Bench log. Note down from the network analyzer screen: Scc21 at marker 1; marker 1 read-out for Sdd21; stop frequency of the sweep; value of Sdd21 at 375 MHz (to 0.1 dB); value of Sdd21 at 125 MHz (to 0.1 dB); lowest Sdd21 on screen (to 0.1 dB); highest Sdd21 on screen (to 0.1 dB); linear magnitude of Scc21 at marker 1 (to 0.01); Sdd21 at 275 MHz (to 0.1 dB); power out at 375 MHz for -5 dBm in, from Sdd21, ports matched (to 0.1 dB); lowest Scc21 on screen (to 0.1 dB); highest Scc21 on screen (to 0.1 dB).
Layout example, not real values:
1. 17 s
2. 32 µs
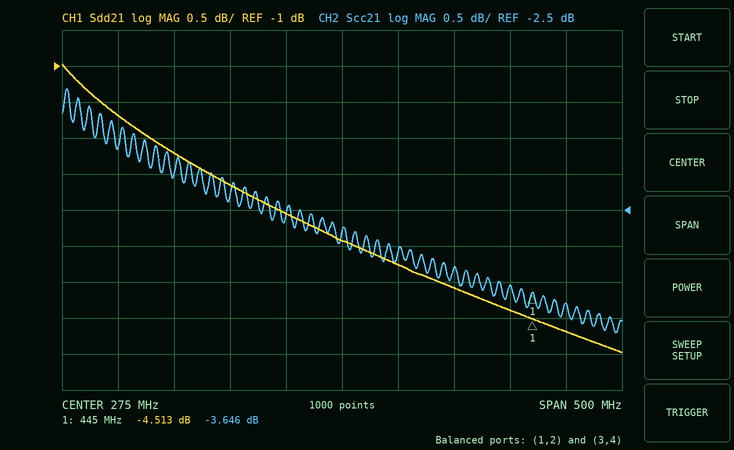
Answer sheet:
1. -3.646 dB
2. -4.513 dB
3. 525 MHz
4. -4.1 dB
5. -2.2 dB
6. -5.0 dB
7. -1.0 dB
8. 0.66
9. -3.4 dB
10. -9.1 dBm
11. -4.2 dB
12. -0.8 dB
